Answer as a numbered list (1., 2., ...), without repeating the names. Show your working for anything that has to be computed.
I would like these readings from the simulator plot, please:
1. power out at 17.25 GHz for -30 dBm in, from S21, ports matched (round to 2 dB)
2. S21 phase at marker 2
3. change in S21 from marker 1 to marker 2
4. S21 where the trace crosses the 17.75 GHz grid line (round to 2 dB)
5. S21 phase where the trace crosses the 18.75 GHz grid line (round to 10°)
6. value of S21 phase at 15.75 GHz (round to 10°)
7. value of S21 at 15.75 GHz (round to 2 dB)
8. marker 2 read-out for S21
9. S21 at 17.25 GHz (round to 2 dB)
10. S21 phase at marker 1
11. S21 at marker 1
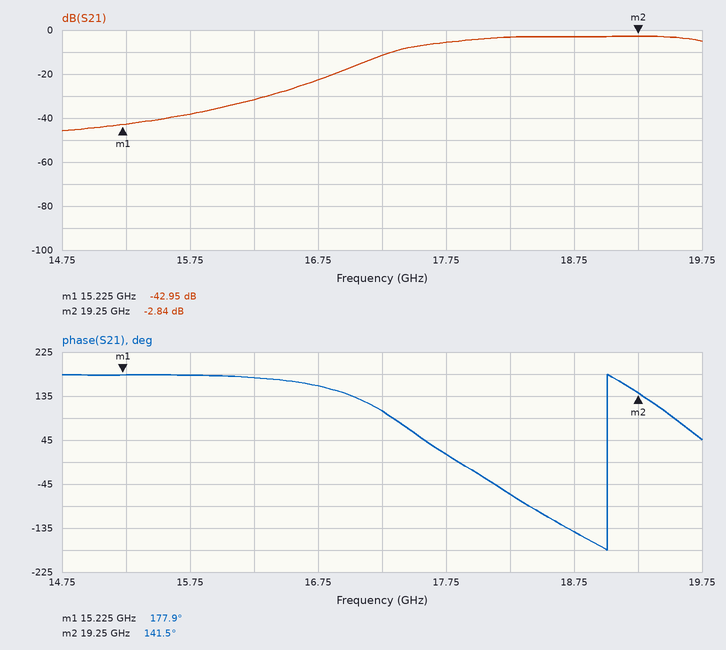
1. -30 dBm + (-12 dB) = -42 dBm
2. 141.5°
3. -2.84 − (-42.95) = 40.11 dB
4. -6 dB
5. -140°
6. 180°
7. -38 dB
8. -2.84 dB
9. -12 dB
10. 177.9°
11. -42.95 dB
